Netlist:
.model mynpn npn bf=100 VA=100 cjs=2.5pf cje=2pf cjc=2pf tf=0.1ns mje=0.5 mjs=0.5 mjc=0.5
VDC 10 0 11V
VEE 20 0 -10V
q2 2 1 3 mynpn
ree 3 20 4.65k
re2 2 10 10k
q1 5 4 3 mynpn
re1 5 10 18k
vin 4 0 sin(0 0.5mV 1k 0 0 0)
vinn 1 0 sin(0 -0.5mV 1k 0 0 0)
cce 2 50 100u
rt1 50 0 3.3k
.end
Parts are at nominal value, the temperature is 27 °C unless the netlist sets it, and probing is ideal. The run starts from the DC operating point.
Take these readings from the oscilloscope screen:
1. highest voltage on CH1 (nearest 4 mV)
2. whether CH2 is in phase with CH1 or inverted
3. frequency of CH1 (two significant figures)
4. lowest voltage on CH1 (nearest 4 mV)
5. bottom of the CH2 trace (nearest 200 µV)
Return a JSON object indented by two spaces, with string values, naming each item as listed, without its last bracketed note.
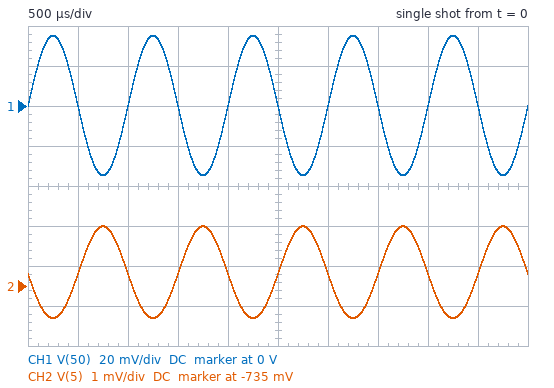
{
  "highest voltage on CH1": "36 mV",
  "whether CH2 is in phase with CH1 or inverted": "inverted",
  "frequency of CH1": "1.0 kHz",
  "lowest voltage on CH1": "-36 mV",
  "bottom of the CH2 trace": "-735.8 mV"
}
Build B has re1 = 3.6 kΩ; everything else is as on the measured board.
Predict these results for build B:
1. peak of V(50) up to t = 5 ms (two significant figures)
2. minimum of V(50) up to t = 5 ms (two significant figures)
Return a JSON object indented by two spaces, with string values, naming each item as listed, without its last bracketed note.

{
  "peak of V(50) up to t = 5 ms": "46 mV",
  "minimum of V(50) up to t = 5 ms": "-46 mV"
}
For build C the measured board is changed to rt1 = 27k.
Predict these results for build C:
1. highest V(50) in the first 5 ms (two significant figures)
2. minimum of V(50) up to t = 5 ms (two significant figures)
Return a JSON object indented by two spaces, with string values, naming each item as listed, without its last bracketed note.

{
  "highest V(50) in the first 5 ms": "100 mV",
  "minimum of V(50) up to t = 5 ms": "-100 mV"
}
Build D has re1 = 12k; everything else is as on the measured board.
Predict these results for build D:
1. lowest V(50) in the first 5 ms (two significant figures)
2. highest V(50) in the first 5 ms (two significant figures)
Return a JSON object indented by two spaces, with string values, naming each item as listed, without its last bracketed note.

{
  "lowest V(50) in the first 5 ms": "-41 mV",
  "highest V(50) in the first 5 ms": "34 mV"
}
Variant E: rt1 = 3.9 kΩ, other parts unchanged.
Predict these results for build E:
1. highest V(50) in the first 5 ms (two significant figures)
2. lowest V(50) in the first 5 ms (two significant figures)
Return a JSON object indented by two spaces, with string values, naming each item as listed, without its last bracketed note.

{
  "highest V(50) in the first 5 ms": "40 mV",
  "lowest V(50) in the first 5 ms": "-39 mV"
}
